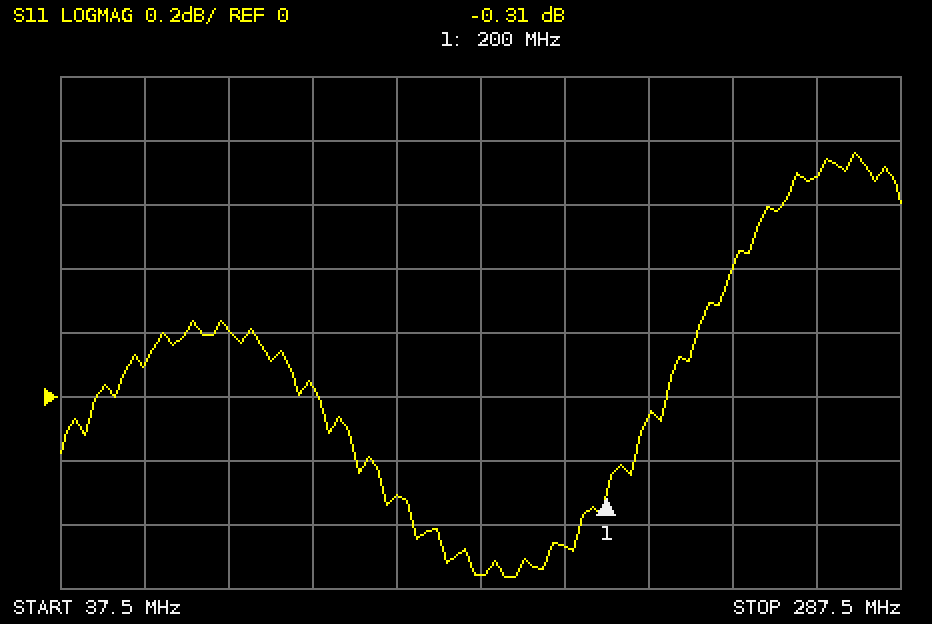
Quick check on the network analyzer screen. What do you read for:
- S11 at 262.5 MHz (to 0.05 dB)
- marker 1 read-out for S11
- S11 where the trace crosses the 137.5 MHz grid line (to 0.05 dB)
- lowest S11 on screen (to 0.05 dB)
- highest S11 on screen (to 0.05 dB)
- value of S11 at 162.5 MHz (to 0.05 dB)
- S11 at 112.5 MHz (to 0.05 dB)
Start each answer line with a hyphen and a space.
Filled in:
- 0.70 dB
- -0.31 dB
- -0.30 dB
- -0.55 dB
- 0.75 dB
- -0.55 dB
- 0.05 dB
